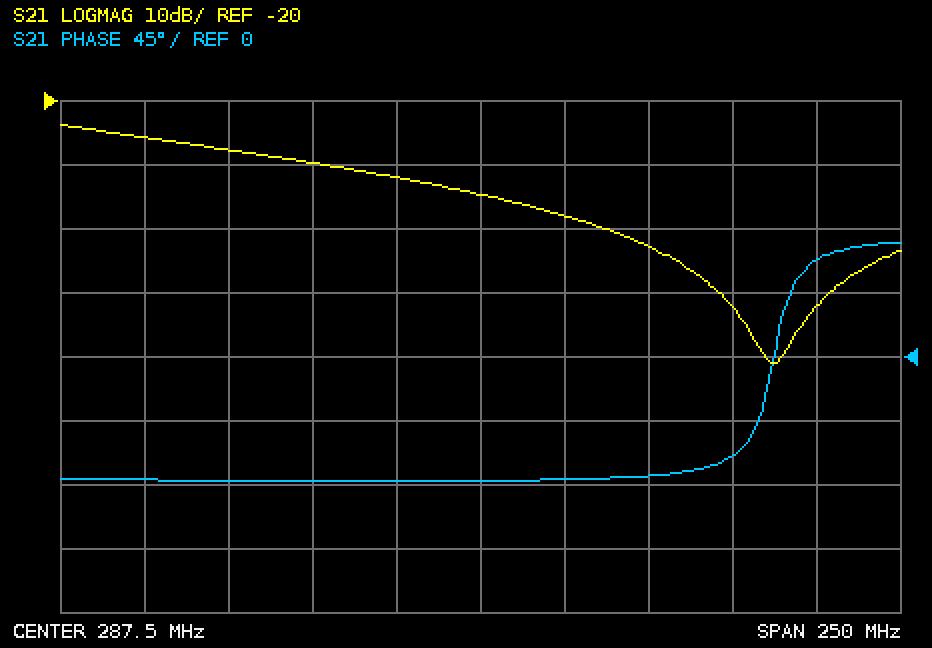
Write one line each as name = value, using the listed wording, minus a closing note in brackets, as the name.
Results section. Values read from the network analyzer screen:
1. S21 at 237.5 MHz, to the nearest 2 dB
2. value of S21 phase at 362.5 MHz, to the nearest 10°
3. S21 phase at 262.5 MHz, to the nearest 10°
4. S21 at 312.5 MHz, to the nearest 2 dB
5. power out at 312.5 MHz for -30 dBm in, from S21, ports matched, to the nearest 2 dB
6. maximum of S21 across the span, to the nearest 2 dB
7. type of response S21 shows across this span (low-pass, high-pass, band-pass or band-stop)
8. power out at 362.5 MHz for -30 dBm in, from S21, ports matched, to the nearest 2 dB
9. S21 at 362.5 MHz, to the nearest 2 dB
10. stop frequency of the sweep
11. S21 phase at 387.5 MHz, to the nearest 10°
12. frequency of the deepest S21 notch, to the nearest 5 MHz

S21 at 237.5 MHz, to the nearest 2 dB = -30 dB
value of S21 phase at 362.5 MHz, to the nearest 10° = -70°
S21 phase at 262.5 MHz, to the nearest 10° = -90°
S21 at 312.5 MHz, to the nearest 2 dB = -38 dB
power out at 312.5 MHz for -30 dBm in, from S21, ports matched, to the nearest 2 dB = -68 dBm
maximum of S21 across the span, to the nearest 2 dB = -24 dB
type of response S21 shows across this span = low-pass
power out at 362.5 MHz for -30 dBm in, from S21, ports matched, to the nearest 2 dB = -82 dBm
S21 at 362.5 MHz, to the nearest 2 dB = -52 dB
stop frequency of the sweep = 412.5 MHz
S21 phase at 387.5 MHz, to the nearest 10° = 70°
frequency of the deepest S21 notch, to the nearest 5 MHz = 375 MHz
